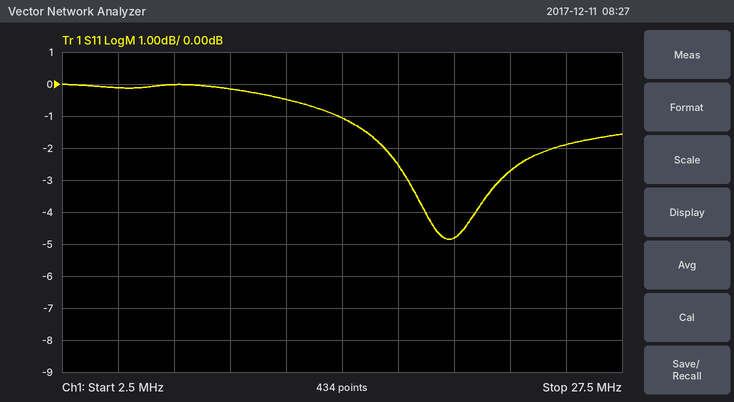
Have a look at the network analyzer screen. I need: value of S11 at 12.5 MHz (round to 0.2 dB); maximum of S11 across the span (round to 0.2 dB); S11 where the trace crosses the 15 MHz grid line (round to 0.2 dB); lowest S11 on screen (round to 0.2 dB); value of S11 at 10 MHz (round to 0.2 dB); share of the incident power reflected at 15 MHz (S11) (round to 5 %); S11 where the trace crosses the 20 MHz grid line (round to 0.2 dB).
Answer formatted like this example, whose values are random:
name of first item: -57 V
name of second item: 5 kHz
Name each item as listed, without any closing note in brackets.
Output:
value of S11 at 12.5 MHz: -0.4 dB
maximum of S11 across the span: 0.0 dB
S11 where the trace crosses the 15 MHz grid line: -1.0 dB
lowest S11 on screen: -4.8 dB
value of S11 at 10 MHz: -0.2 dB
share of the incident power reflected at 15 MHz (S11): 80 %
S11 where the trace crosses the 20 MHz grid line: -4.8 dB
